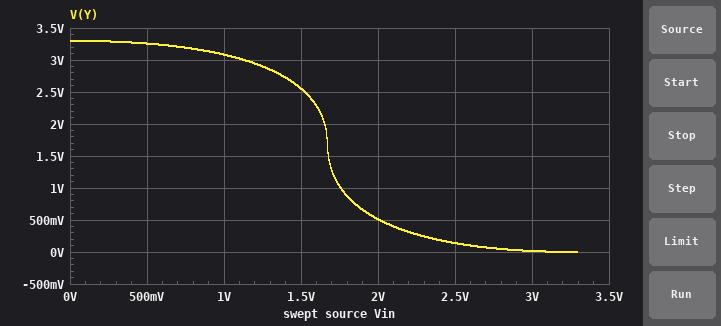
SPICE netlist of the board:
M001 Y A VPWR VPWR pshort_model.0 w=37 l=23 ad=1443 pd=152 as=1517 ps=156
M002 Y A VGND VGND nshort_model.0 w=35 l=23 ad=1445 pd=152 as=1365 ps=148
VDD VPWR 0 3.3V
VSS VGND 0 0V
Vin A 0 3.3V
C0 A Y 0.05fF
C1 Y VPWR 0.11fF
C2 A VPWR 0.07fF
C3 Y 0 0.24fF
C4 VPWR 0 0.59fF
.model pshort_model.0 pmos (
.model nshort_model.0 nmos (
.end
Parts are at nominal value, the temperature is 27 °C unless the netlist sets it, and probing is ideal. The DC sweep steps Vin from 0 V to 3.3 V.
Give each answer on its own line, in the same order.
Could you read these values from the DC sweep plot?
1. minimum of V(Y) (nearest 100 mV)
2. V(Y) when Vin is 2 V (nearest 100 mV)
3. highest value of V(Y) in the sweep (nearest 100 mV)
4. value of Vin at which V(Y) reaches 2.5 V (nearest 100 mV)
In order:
0 V
500 mV
3.3 V
1.5 V
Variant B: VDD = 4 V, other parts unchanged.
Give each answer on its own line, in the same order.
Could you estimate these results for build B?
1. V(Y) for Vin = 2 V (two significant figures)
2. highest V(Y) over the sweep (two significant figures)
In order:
2.5 V
4.0 V
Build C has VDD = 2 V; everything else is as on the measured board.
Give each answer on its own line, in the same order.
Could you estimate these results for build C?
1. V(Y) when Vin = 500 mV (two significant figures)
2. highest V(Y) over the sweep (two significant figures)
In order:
1.9 V
2.0 V
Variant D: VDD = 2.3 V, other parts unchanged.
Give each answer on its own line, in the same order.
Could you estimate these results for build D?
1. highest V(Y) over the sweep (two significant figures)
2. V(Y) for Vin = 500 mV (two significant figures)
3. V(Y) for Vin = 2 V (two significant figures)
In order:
2.3 V
2.2 V
24 mV
